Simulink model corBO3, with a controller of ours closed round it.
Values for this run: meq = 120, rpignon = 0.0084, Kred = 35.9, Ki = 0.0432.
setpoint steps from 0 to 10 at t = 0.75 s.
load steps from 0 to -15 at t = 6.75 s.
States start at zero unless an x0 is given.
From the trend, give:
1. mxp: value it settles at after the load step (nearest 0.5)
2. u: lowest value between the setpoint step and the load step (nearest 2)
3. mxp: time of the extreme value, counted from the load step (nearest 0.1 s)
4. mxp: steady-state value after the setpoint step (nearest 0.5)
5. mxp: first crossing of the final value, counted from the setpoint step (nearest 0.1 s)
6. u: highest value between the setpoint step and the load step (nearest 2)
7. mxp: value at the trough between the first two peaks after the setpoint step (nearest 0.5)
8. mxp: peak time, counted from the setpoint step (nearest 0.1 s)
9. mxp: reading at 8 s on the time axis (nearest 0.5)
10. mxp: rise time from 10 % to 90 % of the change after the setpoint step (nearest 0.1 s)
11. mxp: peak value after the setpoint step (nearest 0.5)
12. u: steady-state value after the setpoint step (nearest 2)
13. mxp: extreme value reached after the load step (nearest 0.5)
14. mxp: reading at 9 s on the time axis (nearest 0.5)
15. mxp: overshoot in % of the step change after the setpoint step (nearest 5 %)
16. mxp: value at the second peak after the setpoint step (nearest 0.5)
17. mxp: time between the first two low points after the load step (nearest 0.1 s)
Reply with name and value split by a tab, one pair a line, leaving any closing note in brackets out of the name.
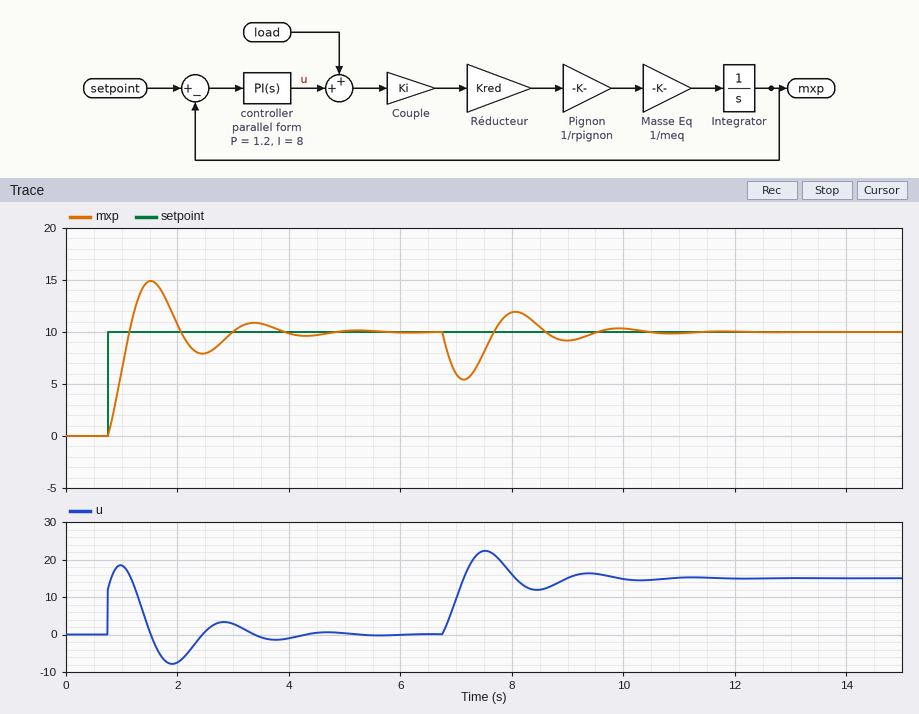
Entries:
mxp: value it settles at after the load step	10.0
u: lowest value between the setpoint step and the load step	-8
mxp: time of the extreme value, counted from the load step	0.4 s
mxp: steady-state value after the setpoint step	10.0
mxp: first crossing of the final value, counted from the setpoint step	0.4 s
u: highest value between the setpoint step and the load step	18
mxp: value at the trough between the first two peaks after the setpoint step	8.0
mxp: peak time, counted from the setpoint step	0.8 s
mxp: reading at 8 s on the time axis	12.0
mxp: rise time from 10 % to 90 % of the change after the setpoint step	0.3 s
mxp: peak value after the setpoint step	15.0
u: steady-state value after the setpoint step	0
mxp: extreme value reached after the load step	5.5
mxp: reading at 9 s on the time axis	9.0
mxp: overshoot in % of the step change after the setpoint step	50 %
mxp: value at the second peak after the setpoint step	11.0
mxp: time between the first two low points after the load step	1.9 s
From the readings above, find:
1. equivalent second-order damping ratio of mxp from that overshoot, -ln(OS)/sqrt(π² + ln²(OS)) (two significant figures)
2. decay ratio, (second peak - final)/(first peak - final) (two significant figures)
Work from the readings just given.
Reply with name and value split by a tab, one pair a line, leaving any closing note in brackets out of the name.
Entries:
equivalent second-order damping ratio of mxp from that overshoot, -ln(OS)/sqrt(π² + ln²(OS))	0.22
decay ratio, (second peak - final)/(first peak - final)	0.20
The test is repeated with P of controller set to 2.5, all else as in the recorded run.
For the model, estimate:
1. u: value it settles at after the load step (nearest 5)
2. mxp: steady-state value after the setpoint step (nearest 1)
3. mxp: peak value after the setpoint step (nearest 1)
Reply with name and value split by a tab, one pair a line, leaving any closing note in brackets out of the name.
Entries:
u: value it settles at after the load step	15
mxp: steady-state value after the setpoint step	10
mxp: peak value after the setpoint step	13
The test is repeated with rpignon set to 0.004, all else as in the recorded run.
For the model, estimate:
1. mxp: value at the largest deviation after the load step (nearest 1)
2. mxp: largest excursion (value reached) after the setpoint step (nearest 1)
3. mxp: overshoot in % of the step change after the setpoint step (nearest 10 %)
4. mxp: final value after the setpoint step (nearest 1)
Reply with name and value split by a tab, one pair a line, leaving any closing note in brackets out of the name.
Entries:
mxp: value at the largest deviation after the load step	4
mxp: largest excursion (value reached) after the setpoint step	14
mxp: overshoot in % of the step change after the setpoint step	40 %
mxp: final value after the setpoint step	10
